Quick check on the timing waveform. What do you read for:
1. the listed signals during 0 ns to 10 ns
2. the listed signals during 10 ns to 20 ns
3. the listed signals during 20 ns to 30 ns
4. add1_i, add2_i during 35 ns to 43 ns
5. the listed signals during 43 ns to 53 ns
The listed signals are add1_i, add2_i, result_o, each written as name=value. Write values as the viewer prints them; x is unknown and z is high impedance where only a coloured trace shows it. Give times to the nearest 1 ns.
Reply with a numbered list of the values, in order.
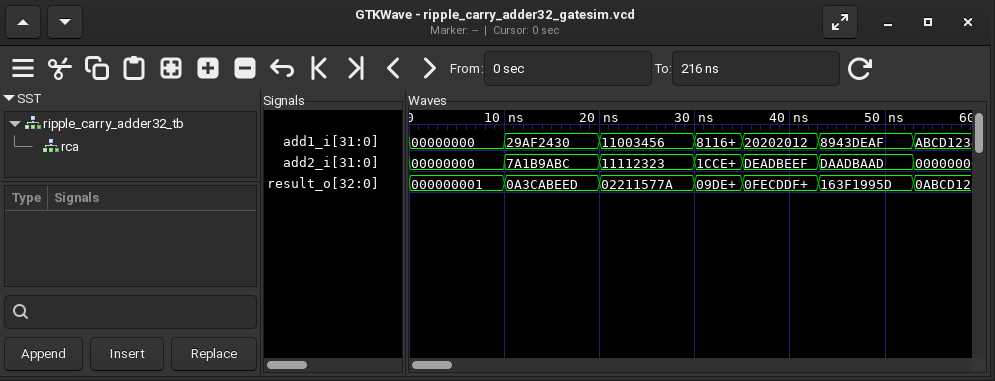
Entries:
1. add1_i=00000000, add2_i=00000000, result_o=000000001
2. add1_i=29AF2430, add2_i=7A1B9ABC, result_o=0A3CABEED
3. add1_i=11003456, add2_i=11112323, result_o=02211577A
4. add1_i=20202012, add2_i=DEADBEEF
5. add1_i=8943DEAF, add2_i=DAADBAAD, result_o=163F1995D
